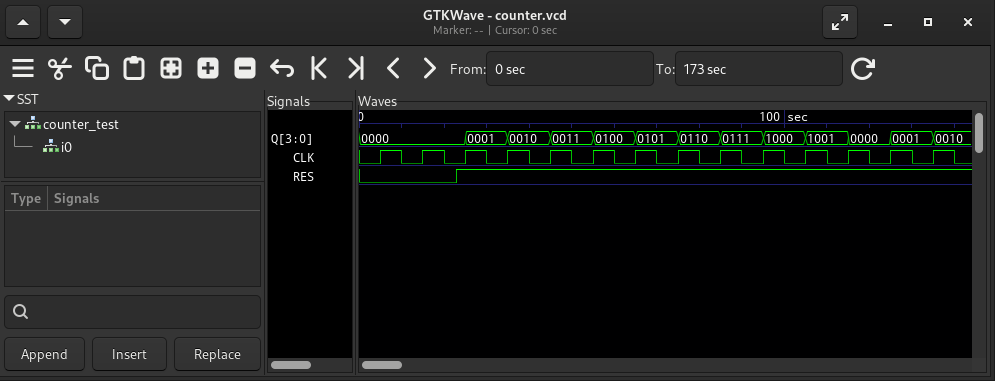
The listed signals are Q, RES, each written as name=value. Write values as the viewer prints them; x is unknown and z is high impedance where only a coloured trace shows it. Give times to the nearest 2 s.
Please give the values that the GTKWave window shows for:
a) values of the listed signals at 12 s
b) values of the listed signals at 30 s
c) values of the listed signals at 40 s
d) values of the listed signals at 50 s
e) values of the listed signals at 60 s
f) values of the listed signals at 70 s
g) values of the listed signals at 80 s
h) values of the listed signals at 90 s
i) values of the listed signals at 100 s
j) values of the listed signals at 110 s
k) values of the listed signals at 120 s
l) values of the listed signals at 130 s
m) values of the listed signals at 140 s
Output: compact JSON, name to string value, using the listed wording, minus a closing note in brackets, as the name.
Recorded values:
{"values of the listed signals at 12 s": "Q=0000, RES=0", "values of the listed signals at 30 s": "Q=0001, RES=1", "values of the listed signals at 40 s": "Q=0010, RES=1", "values of the listed signals at 50 s": "Q=0011, RES=1", "values of the listed signals at 60 s": "Q=0100, RES=1", "values of the listed signals at 70 s": "Q=0101, RES=1", "values of the listed signals at 80 s": "Q=0110, RES=1", "values of the listed signals at 90 s": "Q=0111, RES=1", "values of the listed signals at 100 s": "Q=1000, RES=1", "values of the listed signals at 110 s": "Q=1001, RES=1", "values of the listed signals at 120 s": "Q=0000, RES=1", "values of the listed signals at 130 s": "Q=0001, RES=1", "values of the listed signals at 140 s": "Q=0010, RES=1"}
